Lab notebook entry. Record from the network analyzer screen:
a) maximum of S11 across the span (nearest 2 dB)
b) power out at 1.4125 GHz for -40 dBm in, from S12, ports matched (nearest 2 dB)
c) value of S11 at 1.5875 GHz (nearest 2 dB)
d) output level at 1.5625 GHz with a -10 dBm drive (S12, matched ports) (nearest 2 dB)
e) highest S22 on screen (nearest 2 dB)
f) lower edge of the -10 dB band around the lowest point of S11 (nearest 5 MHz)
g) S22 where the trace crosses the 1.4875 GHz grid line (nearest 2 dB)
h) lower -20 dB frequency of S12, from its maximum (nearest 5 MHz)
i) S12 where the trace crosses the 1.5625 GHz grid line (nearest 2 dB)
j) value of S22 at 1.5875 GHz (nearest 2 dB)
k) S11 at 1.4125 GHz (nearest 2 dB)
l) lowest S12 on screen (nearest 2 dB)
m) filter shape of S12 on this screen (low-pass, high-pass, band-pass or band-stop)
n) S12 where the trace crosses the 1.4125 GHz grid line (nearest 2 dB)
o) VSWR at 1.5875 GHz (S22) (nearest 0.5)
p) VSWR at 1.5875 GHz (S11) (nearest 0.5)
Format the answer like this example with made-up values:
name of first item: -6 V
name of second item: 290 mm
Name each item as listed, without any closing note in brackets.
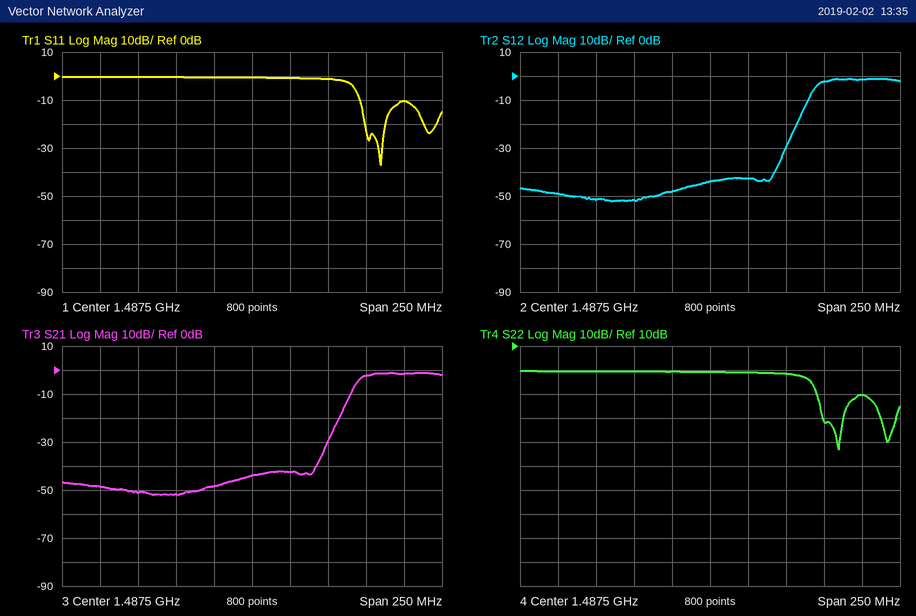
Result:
maximum of S11 across the span: 0 dB
power out at 1.4125 GHz for -40 dBm in, from S12, ports matched: -92 dBm
value of S11 at 1.5875 GHz: -10 dB
output level at 1.5625 GHz with a -10 dBm drive (S12, matched ports): -12 dBm
highest S22 on screen: 0 dB
lower edge of the -10 dB band around the lowest point of S11: 1.560 GHz
S22 where the trace crosses the 1.4875 GHz grid line: 0 dB
lower -20 dB frequency of S12, from its maximum: 1.545 GHz
S12 where the trace crosses the 1.5625 GHz grid line: -2 dB
value of S22 at 1.5875 GHz: -10 dB
S11 at 1.4125 GHz: 0 dB
lowest S12 on screen: -52 dB
filter shape of S12 on this screen: high-pass
S12 where the trace crosses the 1.4125 GHz grid line: -52 dB
VSWR at 1.5875 GHz (S22): 2.0
VSWR at 1.5875 GHz (S11): 2.0
